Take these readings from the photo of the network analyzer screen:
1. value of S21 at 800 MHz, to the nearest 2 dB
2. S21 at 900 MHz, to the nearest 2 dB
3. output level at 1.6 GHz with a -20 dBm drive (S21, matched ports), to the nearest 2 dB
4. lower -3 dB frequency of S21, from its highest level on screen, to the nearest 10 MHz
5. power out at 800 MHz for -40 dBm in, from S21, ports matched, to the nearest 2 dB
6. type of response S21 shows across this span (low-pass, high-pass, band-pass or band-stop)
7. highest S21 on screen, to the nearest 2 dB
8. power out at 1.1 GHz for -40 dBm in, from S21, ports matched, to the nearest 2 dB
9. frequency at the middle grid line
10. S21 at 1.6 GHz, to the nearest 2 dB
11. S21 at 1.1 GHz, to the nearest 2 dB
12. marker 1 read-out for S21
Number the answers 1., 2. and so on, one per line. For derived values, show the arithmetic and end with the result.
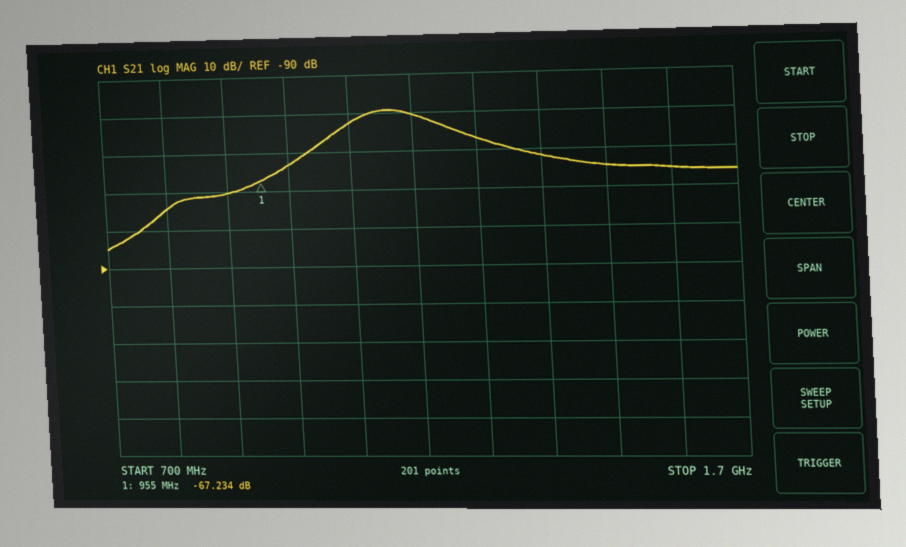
1. -74 dB
2. -70 dB
3. -20 dBm + (-66 dB) = -86 dBm
4. 1.10 GHz
5. -40 dBm + (-74 dB) = -114 dBm
6. band-pass
7. -50 dB
8. -40 dBm + (-52 dB) = -92 dBm
9. 1.2 GHz
10. -66 dB
11. -52 dB
12. -67.234 dB
